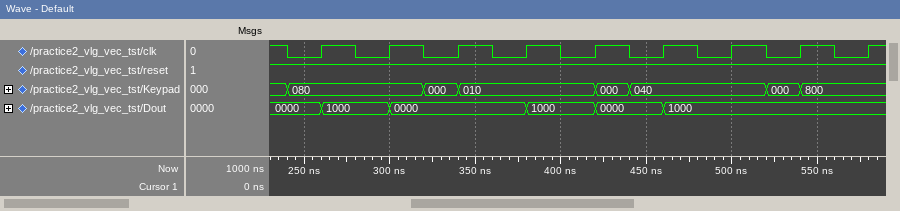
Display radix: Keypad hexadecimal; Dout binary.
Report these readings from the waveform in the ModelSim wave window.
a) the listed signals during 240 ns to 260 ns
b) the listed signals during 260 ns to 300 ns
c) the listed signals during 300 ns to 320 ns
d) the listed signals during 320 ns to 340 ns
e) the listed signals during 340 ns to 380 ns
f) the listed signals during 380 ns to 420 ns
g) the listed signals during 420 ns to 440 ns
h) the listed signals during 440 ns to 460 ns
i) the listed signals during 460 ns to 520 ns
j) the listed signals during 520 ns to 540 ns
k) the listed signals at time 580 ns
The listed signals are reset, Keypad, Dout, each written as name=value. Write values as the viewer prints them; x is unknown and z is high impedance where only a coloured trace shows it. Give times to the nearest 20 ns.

reset=1, Keypad=080, Dout=0000
reset=1, Keypad=080, Dout=1000
reset=1, Keypad=080, Dout=0000
reset=1, Keypad=000, Dout=0000
reset=1, Keypad=010, Dout=0000
reset=1, Keypad=010, Dout=1000
reset=1, Keypad=000, Dout=0000
reset=1, Keypad=040, Dout=0000
reset=1, Keypad=040, Dout=1000
reset=1, Keypad=000, Dout=1000
reset=1, Keypad=800, Dout=1000
